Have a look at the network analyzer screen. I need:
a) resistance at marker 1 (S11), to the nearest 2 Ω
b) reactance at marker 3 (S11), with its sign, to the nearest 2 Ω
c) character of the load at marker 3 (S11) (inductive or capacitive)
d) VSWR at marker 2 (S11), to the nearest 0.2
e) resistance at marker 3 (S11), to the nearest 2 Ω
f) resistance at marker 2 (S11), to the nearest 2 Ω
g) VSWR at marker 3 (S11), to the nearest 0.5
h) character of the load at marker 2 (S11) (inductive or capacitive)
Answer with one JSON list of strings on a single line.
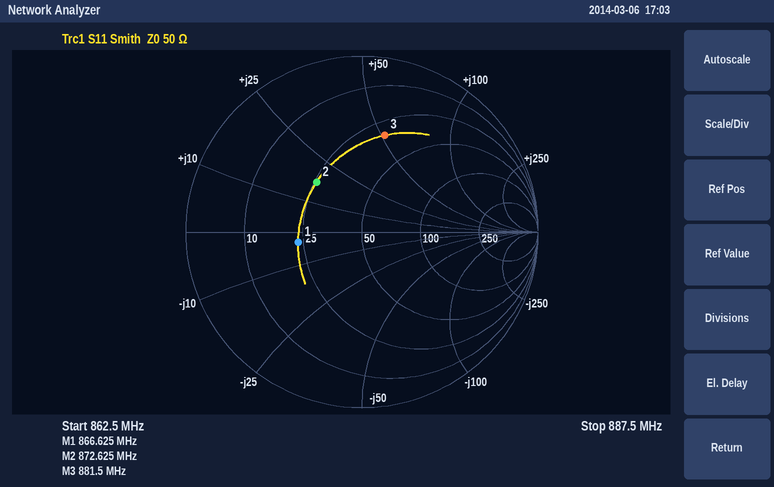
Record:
["24 Ω", "+52 Ω", "inductive", "2.2", "32 Ω", "26 Ω", "3.5", "inductive"]
